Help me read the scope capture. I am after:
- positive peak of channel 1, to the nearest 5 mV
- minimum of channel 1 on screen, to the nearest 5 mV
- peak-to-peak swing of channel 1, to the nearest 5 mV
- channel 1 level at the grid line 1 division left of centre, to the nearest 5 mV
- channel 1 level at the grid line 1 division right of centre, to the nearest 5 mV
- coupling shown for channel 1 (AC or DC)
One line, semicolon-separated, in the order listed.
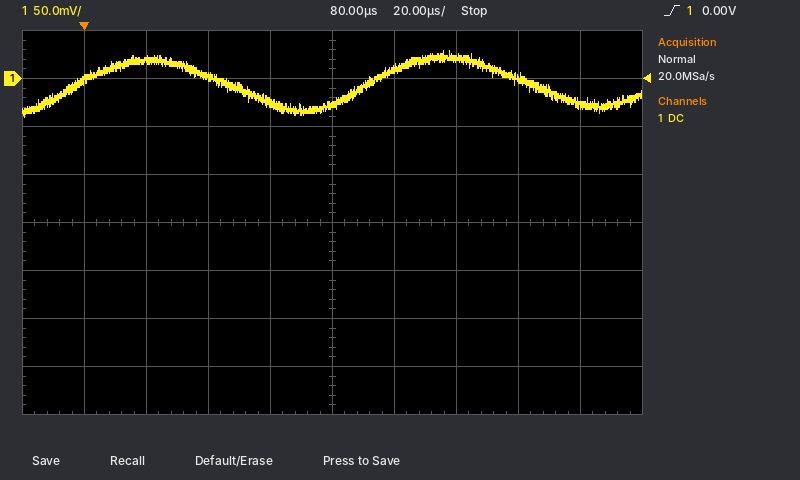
30 mV; -40 mV; 70 mV; -25 mV; 10 mV; DC
